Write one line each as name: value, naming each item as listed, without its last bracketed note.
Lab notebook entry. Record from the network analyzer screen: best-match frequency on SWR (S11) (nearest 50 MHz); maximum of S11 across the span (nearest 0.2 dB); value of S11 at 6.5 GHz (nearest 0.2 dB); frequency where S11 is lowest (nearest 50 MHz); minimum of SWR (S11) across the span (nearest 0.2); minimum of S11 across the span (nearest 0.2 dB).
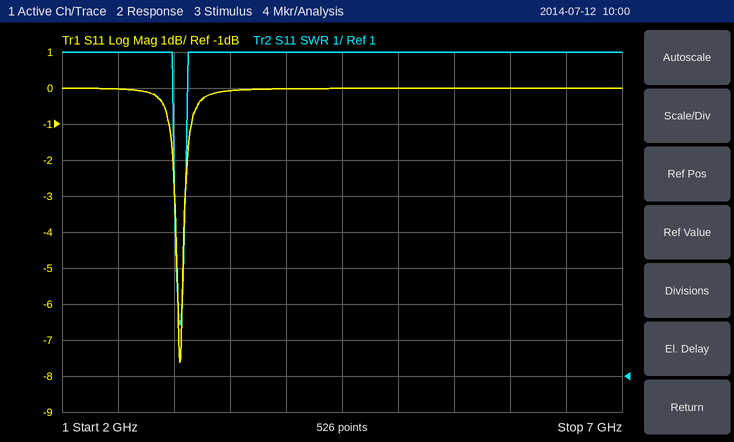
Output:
best-match frequency on SWR (S11): 3.05 GHz
maximum of S11 across the span: 0.0 dB
value of S11 at 6.5 GHz: 0.0 dB
frequency where S11 is lowest: 3.05 GHz
minimum of SWR (S11) across the span: 2.4
minimum of S11 across the span: -7.6 dB
